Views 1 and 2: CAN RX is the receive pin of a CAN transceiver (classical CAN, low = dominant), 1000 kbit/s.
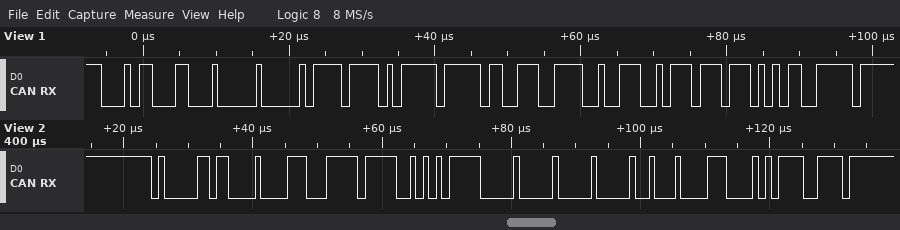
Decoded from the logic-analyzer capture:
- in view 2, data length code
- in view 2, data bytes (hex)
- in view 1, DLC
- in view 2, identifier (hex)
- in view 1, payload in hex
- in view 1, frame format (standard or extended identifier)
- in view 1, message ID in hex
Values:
8
71 FF AA F8 00 00 22 1C
8
0x416
00 F7 AF FF 39 E4 E5 DD
standard
0x163
